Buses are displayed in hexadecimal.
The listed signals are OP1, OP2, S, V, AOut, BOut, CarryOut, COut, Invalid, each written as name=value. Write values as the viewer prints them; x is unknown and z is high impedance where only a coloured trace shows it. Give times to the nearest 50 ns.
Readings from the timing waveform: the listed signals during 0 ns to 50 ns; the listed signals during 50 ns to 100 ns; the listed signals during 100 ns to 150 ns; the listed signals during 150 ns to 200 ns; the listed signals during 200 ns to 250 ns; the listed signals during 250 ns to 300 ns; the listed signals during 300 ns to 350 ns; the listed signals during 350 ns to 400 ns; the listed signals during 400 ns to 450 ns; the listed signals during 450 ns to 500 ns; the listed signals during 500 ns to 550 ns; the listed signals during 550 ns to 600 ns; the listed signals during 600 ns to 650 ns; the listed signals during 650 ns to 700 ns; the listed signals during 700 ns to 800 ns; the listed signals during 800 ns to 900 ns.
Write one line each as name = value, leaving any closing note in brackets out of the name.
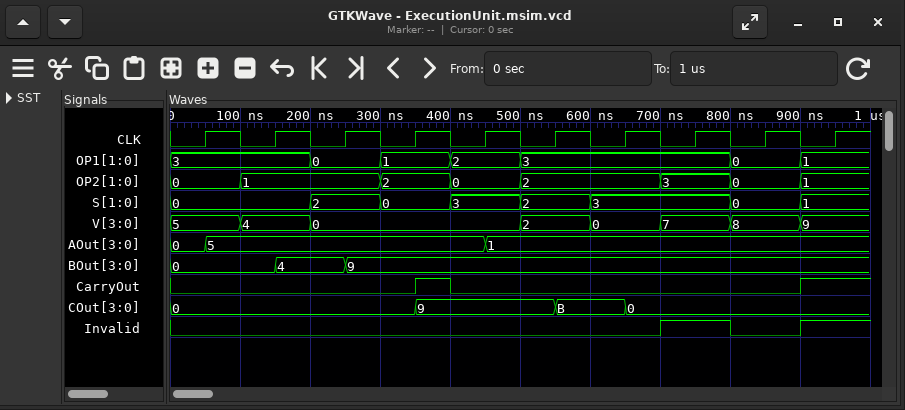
the listed signals during 0 ns to 50 ns = OP1=3, OP2=0, S=0, V=5, AOut=0, BOut=0, CarryOut=0, COut=0, Invalid=0
the listed signals during 50 ns to 100 ns = OP1=3, OP2=0, S=0, V=5, AOut=5, BOut=0, CarryOut=0, COut=0, Invalid=0
the listed signals during 100 ns to 150 ns = OP1=3, OP2=1, S=0, V=4, AOut=5, BOut=0, CarryOut=0, COut=0, Invalid=0
the listed signals during 150 ns to 200 ns = OP1=3, OP2=1, S=0, V=4, AOut=5, BOut=4, CarryOut=0, COut=0, Invalid=0
the listed signals during 200 ns to 250 ns = OP1=0, OP2=1, S=2, V=0, AOut=5, BOut=4, CarryOut=0, COut=0, Invalid=0
the listed signals during 250 ns to 300 ns = OP1=0, OP2=1, S=2, V=0, AOut=5, BOut=9, CarryOut=0, COut=0, Invalid=0
the listed signals during 300 ns to 350 ns = OP1=1, OP2=2, S=0, V=0, AOut=5, BOut=9, CarryOut=0, COut=0, Invalid=0
the listed signals during 350 ns to 400 ns = OP1=1, OP2=2, S=0, V=0, AOut=5, BOut=9, CarryOut=1, COut=9, Invalid=0
the listed signals during 400 ns to 450 ns = OP1=2, OP2=0, S=3, V=0, AOut=5, BOut=9, CarryOut=0, COut=9, Invalid=0
the listed signals during 450 ns to 500 ns = OP1=2, OP2=0, S=3, V=0, AOut=1, BOut=9, CarryOut=0, COut=9, Invalid=0
the listed signals during 500 ns to 550 ns = OP1=3, OP2=2, S=2, V=2, AOut=1, BOut=9, CarryOut=0, COut=9, Invalid=0
the listed signals during 550 ns to 600 ns = OP1=3, OP2=2, S=2, V=2, AOut=1, BOut=9, CarryOut=0, COut=B, Invalid=0
the listed signals during 600 ns to 650 ns = OP1=3, OP2=2, S=3, V=0, AOut=1, BOut=9, CarryOut=0, COut=B, Invalid=0
the listed signals during 650 ns to 700 ns = OP1=3, OP2=2, S=3, V=0, AOut=1, BOut=9, CarryOut=0, COut=0, Invalid=0
the listed signals during 700 ns to 800 ns = OP1=3, OP2=3, S=3, V=7, AOut=1, BOut=9, CarryOut=0, COut=0, Invalid=1
the listed signals during 800 ns to 900 ns = OP1=0, OP2=0, S=0, V=8, AOut=1, BOut=9, CarryOut=0, COut=0, Invalid=0
